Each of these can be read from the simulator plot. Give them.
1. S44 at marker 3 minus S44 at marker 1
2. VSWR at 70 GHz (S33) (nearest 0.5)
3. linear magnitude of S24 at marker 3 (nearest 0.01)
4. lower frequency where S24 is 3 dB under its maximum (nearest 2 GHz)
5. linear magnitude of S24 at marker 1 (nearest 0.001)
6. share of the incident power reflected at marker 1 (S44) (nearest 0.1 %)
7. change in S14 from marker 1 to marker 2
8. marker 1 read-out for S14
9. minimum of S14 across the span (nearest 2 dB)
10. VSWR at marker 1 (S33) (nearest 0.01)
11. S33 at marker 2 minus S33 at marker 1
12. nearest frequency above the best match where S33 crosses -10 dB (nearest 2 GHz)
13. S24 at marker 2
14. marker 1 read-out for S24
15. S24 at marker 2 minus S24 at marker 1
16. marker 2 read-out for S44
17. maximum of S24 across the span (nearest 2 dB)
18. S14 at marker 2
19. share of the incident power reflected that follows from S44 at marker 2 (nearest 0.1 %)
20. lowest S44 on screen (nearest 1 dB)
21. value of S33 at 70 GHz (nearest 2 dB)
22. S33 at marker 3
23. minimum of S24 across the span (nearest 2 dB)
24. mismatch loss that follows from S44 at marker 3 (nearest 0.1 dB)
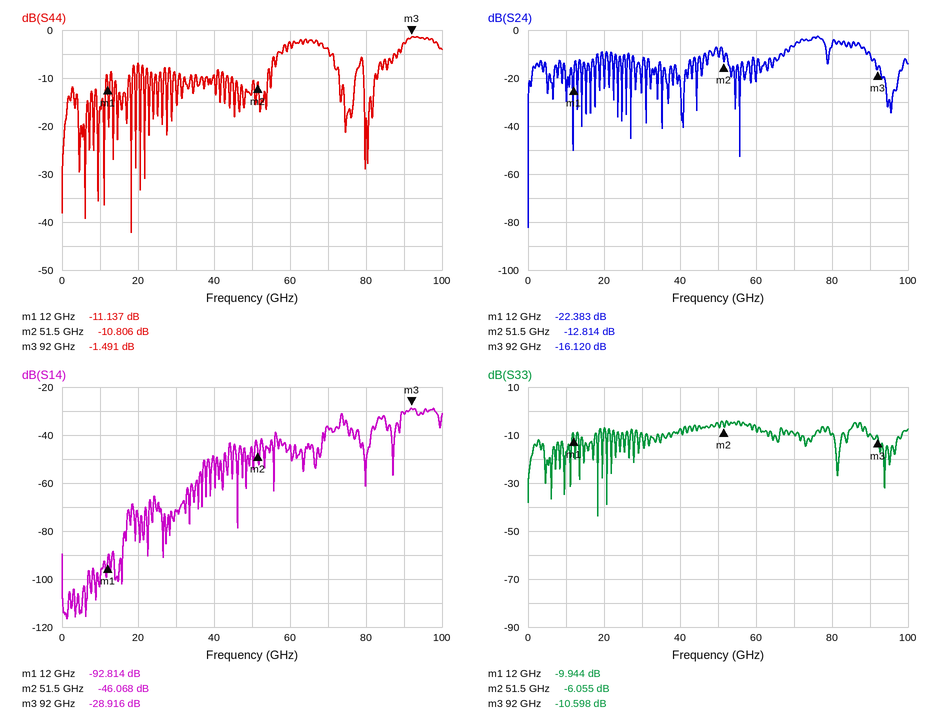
9.646 dB
2.0
0.16
70 GHz
0.076
7.7 %
46.746 dB
-92.814 dB
-116 dB
1.93
3.889 dB
18 GHz
-12.814 dB
-22.383 dB
9.569 dB
-10.806 dB
-2 dB
-46.068 dB
8.3 %
-42 dB
-10 dB
-10.598 dB
-82 dB
5.4 dB
